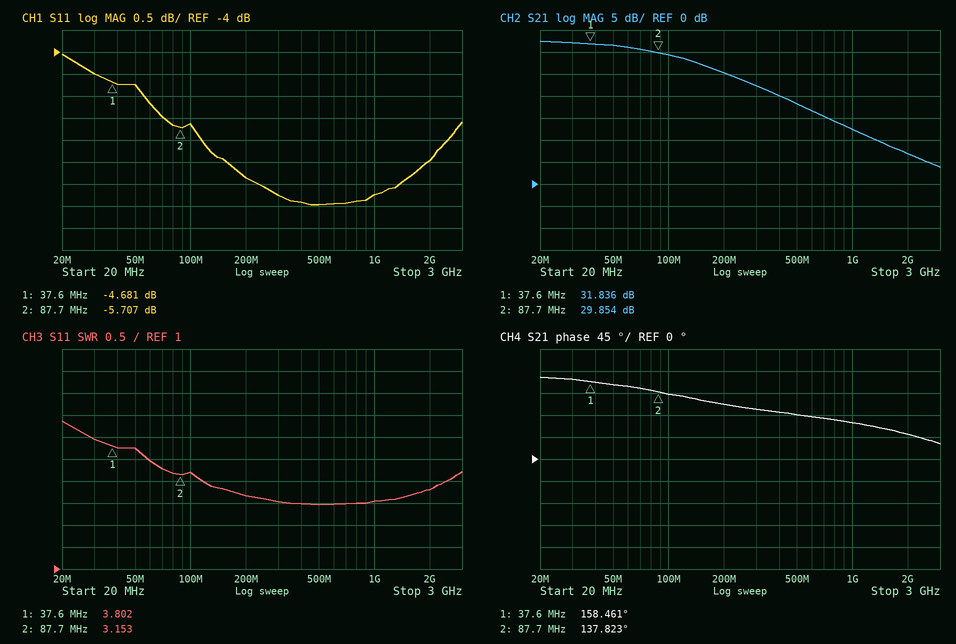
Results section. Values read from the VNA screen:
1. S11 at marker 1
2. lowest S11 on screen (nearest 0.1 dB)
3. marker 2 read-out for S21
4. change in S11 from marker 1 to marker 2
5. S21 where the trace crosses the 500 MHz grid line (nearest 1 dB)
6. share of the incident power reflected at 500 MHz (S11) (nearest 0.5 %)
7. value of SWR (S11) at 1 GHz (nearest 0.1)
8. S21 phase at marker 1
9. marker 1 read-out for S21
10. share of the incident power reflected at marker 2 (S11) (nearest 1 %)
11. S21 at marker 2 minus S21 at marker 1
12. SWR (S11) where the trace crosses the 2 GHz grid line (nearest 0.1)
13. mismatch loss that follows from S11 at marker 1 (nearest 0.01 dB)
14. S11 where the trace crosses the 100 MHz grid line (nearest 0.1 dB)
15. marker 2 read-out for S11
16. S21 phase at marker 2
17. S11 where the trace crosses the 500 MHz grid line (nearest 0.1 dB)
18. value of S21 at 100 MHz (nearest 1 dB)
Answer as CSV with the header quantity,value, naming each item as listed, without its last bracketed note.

quantity,value
S11 at marker 1,-4.681 dB
lowest S11 on screen,-7.5 dB
marker 2 read-out for S21,29.854 dB
change in S11 from marker 1 to marker 2,-1.026 dB
S21 where the trace crosses the 500 MHz grid line,18 dB
share of the incident power reflected at 500 MHz (S11),18.0 %
value of SWR (S11) at 1 GHz,2.5
S21 phase at marker 1,158.461°
marker 1 read-out for S21,31.836 dB
share of the incident power reflected at marker 2 (S11),27 %
S21 at marker 2 minus S21 at marker 1,-1.982 dB
SWR (S11) where the trace crosses the 2 GHz grid line,2.8
mismatch loss that follows from S11 at marker 1,1.81 dB
S11 where the trace crosses the 100 MHz grid line,-5.6 dB
marker 2 read-out for S11,-5.707 dB
S21 phase at marker 2,137.823°
S11 where the trace crosses the 500 MHz grid line,-7.5 dB
value of S21 at 100 MHz,29 dB
